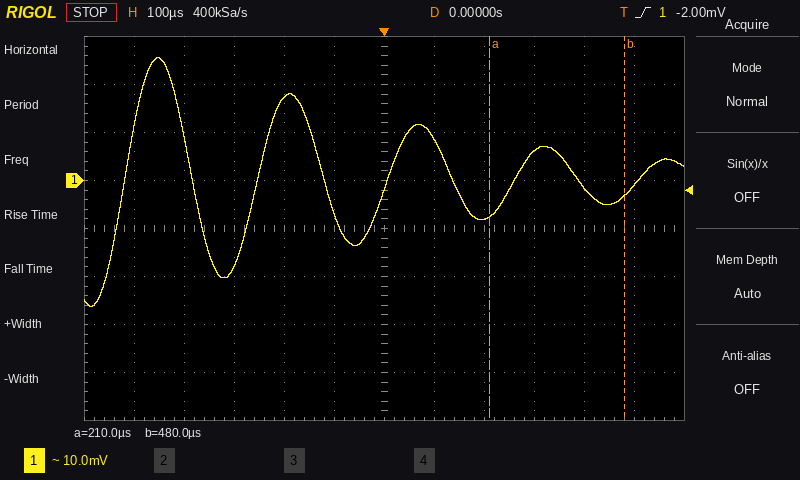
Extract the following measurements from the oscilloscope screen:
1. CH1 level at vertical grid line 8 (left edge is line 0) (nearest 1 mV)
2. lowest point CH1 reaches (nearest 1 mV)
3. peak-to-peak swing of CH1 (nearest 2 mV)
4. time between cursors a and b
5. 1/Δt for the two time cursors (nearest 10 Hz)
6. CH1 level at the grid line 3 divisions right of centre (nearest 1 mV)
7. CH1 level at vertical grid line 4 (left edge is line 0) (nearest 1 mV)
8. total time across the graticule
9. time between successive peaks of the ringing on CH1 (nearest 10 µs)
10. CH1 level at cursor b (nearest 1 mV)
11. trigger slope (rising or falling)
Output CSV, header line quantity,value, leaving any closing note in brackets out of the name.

quantity,value
CH1 level at vertical grid line 8 (left edge is line 0),-8 mV
lowest point CH1 reaches,-26 mV
peak-to-peak swing of CH1,52 mV
time between cursors a and b,270 µs
1/Δt for the two time cursors,3.70 kHz
CH1 level at the grid line 3 divisions right of centre,6 mV
CH1 level at vertical grid line 4 (left edge is line 0),17 mV
total time across the graticule,1.2 ms
time between successive peaks of the ringing on CH1,260 µs
CH1 level at cursor b,-3 mV
trigger slope,rising
